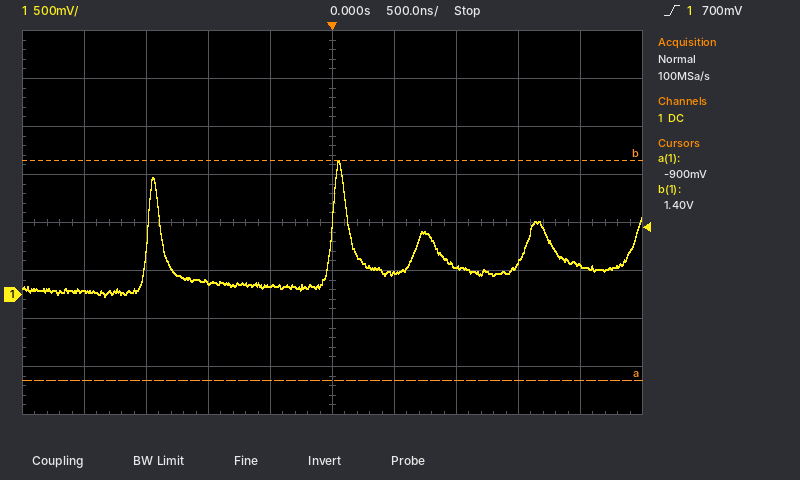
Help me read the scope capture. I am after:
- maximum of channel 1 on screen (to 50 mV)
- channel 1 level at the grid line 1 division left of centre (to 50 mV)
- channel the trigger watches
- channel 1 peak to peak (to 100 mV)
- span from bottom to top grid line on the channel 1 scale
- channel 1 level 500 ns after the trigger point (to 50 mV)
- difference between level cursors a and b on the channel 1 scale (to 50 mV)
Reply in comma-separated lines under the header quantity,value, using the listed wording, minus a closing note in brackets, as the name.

quantity,value
maximum of channel 1 on screen,1.40 V
channel 1 level at the grid line 1 division left of centre,100 mV
channel the trigger watches,channel 1
channel 1 peak to peak,1.40 V
span from bottom to top grid line on the channel 1 scale,4 V
channel 1 level 500 ns after the trigger point,200 mV
difference between level cursors a and b on the channel 1 scale,2.30 V
